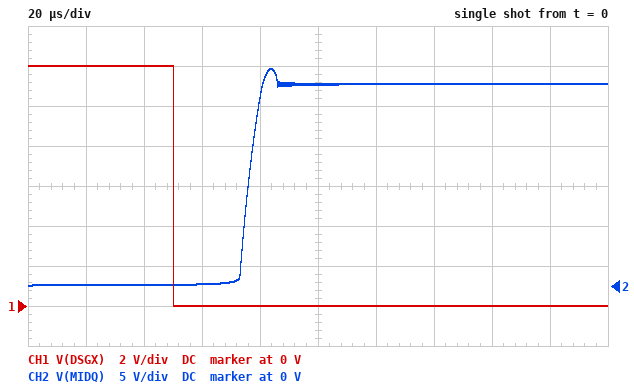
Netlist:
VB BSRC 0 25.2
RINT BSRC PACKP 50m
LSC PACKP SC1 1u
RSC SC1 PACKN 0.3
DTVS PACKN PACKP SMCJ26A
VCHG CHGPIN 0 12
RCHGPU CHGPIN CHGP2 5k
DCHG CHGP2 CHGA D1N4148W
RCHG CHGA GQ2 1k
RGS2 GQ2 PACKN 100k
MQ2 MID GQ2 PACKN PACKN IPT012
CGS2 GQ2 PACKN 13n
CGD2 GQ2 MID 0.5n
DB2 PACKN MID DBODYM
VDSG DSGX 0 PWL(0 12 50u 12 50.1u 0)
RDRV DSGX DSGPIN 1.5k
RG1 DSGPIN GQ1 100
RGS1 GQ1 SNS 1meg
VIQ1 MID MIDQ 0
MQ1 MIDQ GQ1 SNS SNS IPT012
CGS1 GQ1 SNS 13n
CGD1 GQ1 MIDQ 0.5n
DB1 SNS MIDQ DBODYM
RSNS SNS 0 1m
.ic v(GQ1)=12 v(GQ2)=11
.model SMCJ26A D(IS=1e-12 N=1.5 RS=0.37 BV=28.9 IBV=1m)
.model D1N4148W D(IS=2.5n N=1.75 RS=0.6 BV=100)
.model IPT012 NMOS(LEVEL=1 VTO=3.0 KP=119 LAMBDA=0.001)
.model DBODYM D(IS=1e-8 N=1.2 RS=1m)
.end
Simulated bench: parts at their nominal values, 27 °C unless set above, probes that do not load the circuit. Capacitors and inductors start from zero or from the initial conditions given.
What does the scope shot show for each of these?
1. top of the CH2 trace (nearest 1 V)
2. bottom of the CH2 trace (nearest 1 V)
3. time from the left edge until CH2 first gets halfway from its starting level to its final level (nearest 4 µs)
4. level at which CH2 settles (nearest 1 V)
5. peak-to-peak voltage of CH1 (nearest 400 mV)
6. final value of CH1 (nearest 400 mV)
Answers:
27 V
0 V
76 µs
25 V
12.0 V
0 V
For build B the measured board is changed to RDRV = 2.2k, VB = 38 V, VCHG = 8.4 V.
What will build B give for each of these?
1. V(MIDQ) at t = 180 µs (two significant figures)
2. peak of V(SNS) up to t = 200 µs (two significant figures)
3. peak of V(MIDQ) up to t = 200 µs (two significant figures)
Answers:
38 V
110 mV
39 V
